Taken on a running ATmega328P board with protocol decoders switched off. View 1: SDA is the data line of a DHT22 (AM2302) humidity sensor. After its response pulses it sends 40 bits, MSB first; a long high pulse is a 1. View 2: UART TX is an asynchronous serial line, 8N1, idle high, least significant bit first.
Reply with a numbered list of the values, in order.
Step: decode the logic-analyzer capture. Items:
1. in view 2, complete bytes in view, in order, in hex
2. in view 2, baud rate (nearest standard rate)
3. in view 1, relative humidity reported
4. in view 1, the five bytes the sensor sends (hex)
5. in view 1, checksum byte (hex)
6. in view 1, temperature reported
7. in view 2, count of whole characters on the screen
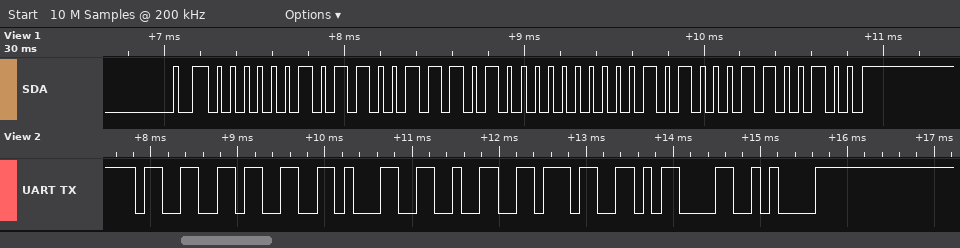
1. 0x33 0x33 0x31 0x32 0x37 0x0D 0x0A
2. 9600 baud
3. 71.8 %
4. 02 CE 80 14 64
5. 0x64
6. -2.0 °C
7. 7
